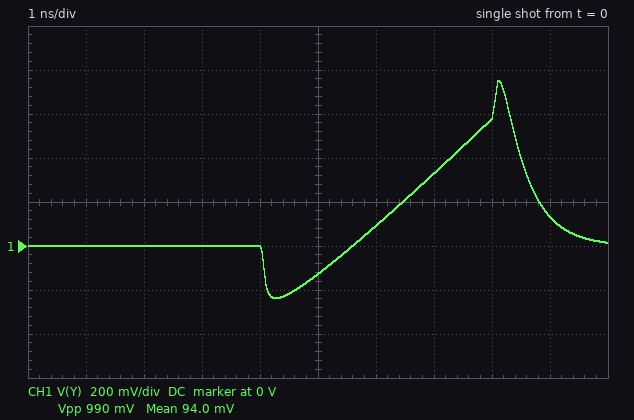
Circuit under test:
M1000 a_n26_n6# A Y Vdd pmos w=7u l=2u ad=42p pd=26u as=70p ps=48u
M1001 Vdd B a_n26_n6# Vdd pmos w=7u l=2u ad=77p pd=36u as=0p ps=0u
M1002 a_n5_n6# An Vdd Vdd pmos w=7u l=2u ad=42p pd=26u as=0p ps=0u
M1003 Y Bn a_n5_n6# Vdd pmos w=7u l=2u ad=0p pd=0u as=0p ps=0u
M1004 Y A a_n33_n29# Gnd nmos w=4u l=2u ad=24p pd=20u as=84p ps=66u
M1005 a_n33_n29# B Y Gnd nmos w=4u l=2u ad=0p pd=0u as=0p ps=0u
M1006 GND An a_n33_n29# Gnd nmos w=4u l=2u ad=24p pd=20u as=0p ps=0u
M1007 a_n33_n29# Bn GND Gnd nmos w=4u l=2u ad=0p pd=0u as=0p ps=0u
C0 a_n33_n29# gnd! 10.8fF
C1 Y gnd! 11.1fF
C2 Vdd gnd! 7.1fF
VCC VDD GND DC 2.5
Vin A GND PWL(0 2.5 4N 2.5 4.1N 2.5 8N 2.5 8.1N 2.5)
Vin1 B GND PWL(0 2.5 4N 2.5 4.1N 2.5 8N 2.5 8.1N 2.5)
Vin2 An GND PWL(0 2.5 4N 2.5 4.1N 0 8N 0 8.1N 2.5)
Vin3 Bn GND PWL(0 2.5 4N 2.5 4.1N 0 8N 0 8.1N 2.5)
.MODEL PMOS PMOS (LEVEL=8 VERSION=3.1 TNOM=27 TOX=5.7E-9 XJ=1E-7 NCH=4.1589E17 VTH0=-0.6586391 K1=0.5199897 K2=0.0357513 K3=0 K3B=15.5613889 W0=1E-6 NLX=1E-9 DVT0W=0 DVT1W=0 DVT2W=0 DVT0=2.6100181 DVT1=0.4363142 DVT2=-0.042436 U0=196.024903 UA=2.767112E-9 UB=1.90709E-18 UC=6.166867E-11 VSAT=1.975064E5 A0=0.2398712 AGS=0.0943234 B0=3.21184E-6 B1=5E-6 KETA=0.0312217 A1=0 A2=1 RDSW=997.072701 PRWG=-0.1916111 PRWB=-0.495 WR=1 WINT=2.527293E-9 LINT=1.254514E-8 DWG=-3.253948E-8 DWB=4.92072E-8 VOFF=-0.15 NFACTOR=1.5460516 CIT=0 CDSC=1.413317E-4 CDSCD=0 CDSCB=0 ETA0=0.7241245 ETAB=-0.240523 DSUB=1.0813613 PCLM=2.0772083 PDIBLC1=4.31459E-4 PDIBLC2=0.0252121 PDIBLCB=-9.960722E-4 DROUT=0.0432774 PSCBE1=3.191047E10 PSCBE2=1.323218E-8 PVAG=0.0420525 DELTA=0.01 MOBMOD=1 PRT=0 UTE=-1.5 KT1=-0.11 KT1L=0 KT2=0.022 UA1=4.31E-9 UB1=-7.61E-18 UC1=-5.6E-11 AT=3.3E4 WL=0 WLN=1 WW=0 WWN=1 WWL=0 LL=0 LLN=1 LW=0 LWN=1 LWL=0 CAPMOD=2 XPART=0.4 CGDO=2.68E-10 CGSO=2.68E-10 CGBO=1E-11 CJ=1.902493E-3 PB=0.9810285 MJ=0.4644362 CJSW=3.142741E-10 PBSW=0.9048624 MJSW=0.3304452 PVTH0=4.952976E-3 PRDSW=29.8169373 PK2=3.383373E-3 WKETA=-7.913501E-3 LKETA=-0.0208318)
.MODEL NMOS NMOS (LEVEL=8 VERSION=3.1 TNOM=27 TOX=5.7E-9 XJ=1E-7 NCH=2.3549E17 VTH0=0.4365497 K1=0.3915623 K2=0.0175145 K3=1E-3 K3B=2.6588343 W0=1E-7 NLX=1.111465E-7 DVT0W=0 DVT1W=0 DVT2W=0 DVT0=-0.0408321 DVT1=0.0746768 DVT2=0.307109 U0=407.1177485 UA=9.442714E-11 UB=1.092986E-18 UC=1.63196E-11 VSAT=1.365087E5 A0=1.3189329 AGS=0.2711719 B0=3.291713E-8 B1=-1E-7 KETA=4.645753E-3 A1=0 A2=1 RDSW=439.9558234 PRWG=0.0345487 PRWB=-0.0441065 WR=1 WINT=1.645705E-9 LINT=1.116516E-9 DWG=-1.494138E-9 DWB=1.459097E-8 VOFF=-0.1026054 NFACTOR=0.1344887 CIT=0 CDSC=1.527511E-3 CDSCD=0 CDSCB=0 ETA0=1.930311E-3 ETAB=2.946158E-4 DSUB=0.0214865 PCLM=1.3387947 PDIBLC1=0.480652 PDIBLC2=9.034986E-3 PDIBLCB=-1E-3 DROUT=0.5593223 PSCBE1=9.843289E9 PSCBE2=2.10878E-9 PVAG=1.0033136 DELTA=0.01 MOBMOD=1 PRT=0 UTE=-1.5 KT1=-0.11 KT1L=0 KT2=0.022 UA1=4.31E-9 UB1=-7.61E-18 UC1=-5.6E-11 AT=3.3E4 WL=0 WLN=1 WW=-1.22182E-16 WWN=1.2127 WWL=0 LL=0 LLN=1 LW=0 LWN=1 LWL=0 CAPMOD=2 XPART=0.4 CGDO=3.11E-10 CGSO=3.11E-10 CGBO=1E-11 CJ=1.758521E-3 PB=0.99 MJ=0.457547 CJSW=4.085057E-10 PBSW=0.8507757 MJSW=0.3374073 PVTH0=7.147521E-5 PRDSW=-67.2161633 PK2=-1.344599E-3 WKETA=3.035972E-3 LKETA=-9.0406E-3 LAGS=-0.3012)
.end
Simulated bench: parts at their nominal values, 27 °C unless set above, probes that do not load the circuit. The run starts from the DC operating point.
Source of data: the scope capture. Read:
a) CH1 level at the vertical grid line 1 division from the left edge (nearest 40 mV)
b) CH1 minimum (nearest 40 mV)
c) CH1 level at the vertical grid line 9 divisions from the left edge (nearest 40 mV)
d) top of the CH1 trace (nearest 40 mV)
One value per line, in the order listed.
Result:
0 V
-240 mV
120 mV
760 mV
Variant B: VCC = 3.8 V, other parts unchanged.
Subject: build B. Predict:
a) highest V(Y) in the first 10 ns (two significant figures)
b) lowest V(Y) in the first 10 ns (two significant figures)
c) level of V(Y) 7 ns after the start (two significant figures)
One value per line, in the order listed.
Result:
2.9 V
-170 mV
1.5 V
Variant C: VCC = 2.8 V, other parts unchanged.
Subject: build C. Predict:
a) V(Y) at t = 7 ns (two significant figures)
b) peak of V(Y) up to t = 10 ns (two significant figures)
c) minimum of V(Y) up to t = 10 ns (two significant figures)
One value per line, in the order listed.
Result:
500 mV
1.0 V
-240 mV
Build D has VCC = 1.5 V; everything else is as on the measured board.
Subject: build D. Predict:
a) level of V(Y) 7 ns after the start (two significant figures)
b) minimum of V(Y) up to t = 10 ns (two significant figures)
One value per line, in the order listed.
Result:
-100 mV
-230 mV
